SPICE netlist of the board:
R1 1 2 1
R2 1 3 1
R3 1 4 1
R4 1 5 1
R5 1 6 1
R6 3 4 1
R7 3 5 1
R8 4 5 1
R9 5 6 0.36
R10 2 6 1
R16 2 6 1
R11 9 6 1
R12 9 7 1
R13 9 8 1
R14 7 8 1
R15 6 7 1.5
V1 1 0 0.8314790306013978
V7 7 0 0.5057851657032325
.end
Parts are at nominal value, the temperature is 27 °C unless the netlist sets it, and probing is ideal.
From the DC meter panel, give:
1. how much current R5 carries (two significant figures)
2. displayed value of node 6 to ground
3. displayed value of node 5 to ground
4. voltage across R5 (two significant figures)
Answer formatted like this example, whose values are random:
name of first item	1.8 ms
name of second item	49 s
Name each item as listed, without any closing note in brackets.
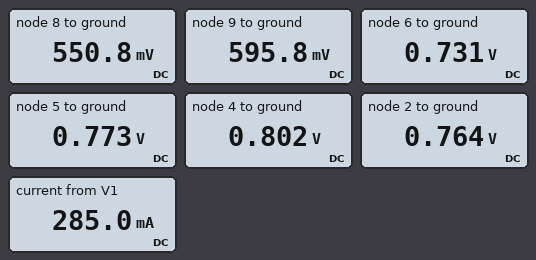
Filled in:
how much current R5 carries	100 mA
displayed value of node 6 to ground	0.731 V
displayed value of node 5 to ground	0.773 V
voltage across R5	100 mV
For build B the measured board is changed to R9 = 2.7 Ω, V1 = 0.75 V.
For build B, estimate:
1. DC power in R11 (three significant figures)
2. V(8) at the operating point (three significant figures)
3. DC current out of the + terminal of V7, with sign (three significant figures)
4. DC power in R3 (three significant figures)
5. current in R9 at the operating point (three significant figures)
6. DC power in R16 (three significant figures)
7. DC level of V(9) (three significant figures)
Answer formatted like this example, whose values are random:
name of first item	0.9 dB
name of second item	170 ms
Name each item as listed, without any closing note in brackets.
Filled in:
DC power in R11	7.98 mW
V(8) at the operating point	536 mV
DC current out of the + terminal of V7, with sign	-189 mA
DC power in R3	55.4 µW
current in R9 at the operating point	29.8 mA
DC power in R16	1.01 mW
DC level of V(9)	565 mV
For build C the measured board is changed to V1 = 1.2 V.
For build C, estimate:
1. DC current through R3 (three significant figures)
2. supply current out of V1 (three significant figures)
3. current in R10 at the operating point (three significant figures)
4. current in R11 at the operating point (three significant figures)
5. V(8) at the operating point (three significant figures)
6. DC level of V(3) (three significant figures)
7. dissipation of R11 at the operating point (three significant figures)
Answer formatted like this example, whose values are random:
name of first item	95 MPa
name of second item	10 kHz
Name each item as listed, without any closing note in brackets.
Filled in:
DC current through R3	62.4 mA
supply current out of V1	607 mA
current in R10 at the operating point	71.6 mA
current in R11 at the operating point	288 mA
V(8) at the operating point	602 mV
DC level of V(3)	1.14 V
dissipation of R11 at the operating point	82.8 mW
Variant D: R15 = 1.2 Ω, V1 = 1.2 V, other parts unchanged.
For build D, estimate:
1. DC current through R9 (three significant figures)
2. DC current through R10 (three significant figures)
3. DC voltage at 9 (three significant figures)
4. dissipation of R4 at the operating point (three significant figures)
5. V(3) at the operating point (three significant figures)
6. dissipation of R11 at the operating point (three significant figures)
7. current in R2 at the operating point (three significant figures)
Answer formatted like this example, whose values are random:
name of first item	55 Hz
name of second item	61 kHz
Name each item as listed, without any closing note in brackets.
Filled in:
DC current through R9	271 mA
DC current through R10	77.8 mA
DC voltage at 9	690 mV
dissipation of R4 at the operating point	18.4 mW
V(3) at the operating point	1.13 V
dissipation of R11 at the operating point	76.4 mW
current in R2 at the operating point	67.9 mA
